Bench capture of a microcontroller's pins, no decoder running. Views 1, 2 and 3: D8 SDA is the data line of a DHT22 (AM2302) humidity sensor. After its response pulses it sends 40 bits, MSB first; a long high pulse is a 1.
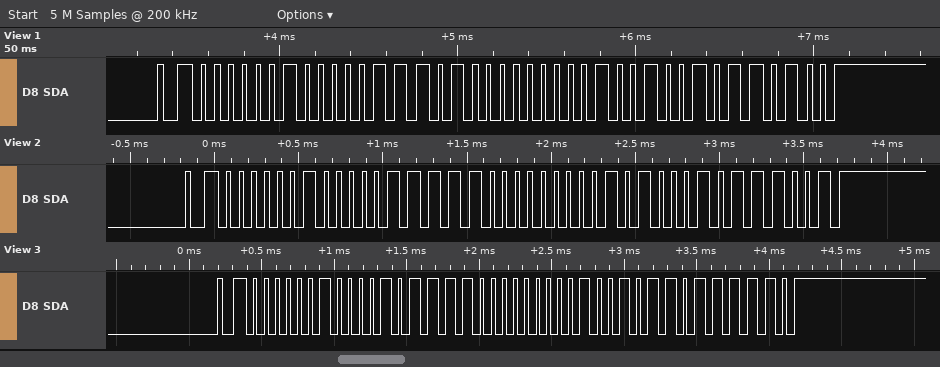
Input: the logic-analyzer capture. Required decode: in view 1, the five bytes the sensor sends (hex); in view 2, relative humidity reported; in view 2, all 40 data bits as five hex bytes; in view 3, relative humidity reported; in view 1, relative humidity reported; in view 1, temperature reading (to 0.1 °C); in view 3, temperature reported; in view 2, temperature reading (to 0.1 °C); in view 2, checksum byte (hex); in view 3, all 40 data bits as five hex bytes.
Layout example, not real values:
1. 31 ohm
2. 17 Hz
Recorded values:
1. 02 0E 80 24 B4
2. 52.7 %
3. 02 0F 80 28 B9
4. 53.5 %
5. 52.6 %
6. -3.6 °C
7. -3.7 °C
8. -4.0 °C
9. 0xB9
10. 02 17 80 25 BE
